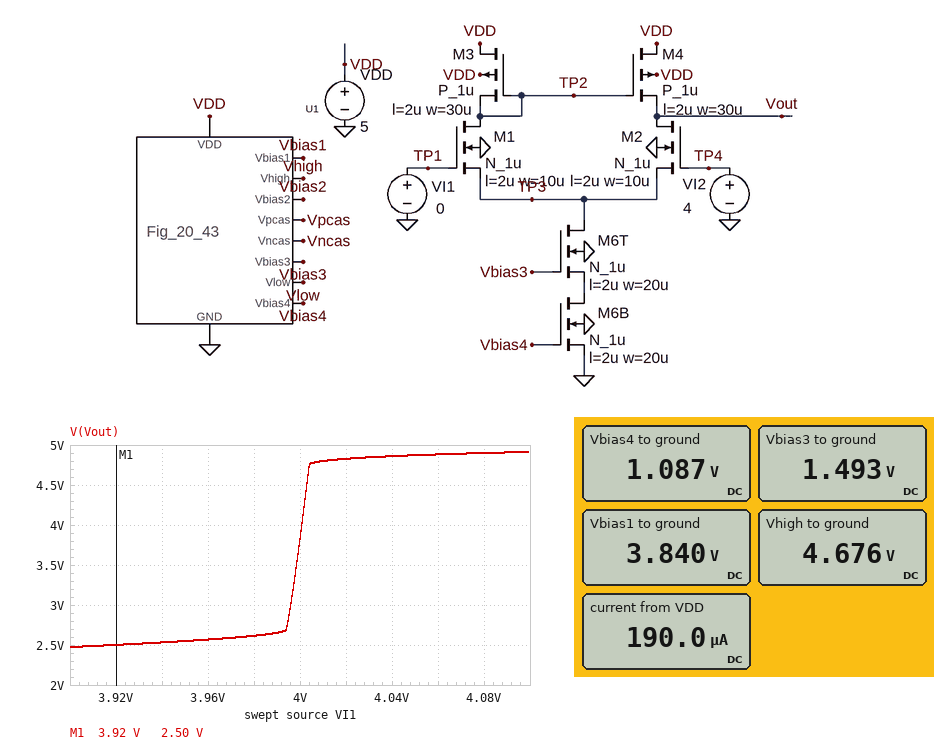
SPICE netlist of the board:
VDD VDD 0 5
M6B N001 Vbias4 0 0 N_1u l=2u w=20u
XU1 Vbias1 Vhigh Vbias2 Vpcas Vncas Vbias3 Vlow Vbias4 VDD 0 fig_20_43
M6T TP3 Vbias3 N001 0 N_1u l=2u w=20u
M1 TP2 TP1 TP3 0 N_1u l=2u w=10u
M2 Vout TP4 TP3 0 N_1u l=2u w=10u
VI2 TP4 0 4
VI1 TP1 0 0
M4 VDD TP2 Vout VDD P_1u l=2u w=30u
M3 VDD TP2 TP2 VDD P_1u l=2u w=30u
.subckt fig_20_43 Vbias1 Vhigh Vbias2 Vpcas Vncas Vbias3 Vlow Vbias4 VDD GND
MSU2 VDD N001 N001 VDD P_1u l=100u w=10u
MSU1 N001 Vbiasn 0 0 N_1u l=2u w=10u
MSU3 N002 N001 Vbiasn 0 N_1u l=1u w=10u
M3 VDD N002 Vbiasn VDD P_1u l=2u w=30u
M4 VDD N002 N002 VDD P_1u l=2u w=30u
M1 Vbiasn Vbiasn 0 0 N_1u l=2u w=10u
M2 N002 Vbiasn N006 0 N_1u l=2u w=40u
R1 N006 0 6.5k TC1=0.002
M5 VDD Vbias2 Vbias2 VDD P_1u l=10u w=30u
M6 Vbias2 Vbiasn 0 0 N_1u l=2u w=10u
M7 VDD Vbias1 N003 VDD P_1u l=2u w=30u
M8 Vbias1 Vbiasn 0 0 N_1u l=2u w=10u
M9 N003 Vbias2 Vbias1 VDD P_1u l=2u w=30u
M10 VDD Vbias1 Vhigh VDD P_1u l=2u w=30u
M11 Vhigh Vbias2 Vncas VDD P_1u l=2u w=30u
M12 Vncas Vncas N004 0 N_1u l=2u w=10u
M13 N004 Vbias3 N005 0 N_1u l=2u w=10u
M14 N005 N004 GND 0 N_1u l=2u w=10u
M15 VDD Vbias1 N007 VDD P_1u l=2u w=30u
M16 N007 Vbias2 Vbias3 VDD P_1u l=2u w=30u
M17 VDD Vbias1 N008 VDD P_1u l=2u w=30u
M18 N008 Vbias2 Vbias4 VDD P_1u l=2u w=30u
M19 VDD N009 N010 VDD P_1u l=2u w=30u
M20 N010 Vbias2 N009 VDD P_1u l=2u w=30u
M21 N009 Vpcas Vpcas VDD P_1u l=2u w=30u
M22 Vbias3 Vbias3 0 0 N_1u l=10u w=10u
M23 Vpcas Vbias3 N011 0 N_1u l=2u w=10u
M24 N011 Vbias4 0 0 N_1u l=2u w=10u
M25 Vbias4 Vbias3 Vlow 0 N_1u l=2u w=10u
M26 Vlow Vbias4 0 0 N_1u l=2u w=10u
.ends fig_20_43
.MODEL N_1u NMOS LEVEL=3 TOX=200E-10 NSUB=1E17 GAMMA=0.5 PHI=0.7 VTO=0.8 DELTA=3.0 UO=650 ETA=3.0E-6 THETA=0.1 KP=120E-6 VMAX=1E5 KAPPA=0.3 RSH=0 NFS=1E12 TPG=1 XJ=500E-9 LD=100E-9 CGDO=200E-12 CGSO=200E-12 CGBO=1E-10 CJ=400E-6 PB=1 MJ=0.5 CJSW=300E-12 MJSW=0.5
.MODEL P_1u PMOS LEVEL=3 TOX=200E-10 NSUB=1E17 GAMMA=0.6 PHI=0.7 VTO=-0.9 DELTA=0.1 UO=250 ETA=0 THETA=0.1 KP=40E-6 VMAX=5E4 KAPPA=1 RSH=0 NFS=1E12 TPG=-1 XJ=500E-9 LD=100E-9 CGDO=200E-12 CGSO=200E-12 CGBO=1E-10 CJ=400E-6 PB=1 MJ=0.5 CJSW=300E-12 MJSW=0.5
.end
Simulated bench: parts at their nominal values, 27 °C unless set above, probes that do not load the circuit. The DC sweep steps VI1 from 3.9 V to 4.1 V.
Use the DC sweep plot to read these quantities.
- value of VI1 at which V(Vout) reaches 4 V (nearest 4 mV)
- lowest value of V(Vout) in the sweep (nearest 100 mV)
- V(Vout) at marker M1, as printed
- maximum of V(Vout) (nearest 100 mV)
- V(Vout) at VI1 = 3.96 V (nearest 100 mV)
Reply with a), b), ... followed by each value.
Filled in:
a) 4.000 V
b) 2.5 V
c) 2.50 V
d) 4.9 V
e) 2.6 V
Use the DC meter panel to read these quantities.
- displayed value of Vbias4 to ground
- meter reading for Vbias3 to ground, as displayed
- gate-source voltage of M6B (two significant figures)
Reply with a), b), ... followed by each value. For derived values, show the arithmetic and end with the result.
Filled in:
a) 1.087 V
b) 1.493 V
c) 1.087 V = 1.1 V
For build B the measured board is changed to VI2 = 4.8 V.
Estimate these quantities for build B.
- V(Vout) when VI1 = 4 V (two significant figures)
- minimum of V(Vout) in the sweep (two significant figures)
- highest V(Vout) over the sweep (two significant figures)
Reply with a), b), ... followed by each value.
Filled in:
a) 2.5 V
b) 2.4 V
c) 2.6 V
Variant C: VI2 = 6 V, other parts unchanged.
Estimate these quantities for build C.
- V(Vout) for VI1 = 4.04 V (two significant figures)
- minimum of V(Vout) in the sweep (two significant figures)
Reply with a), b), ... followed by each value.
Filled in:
a) 2.5 V
b) 2.4 V
